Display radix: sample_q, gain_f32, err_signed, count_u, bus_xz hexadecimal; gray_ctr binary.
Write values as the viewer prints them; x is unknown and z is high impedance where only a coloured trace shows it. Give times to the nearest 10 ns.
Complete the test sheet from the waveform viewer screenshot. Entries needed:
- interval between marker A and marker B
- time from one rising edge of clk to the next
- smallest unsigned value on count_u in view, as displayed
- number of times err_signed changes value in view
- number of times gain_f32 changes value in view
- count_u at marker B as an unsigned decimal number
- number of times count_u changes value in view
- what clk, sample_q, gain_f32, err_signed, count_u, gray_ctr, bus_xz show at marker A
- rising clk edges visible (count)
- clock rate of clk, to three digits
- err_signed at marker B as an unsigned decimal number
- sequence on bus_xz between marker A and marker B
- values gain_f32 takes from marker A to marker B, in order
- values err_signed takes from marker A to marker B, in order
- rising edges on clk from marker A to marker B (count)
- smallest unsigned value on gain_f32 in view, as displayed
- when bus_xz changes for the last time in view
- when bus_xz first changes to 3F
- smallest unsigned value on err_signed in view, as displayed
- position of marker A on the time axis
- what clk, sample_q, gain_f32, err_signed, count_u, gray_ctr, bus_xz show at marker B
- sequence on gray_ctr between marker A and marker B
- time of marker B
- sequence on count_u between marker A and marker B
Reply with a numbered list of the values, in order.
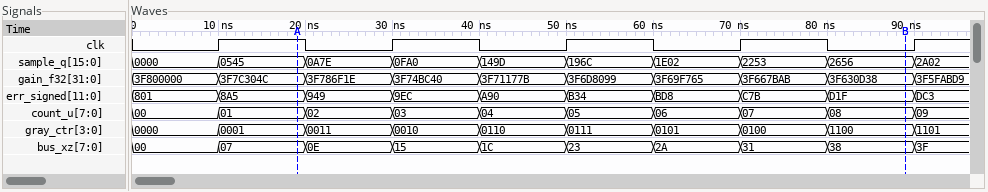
1. 70 ns
2. 20 ns
3. 00
4. 9
5. 9
6. 8
7. 9
8. clk=1, sample_q=0545, gain_f32=3F7C304C, err_signed=8A5, count_u=01, gray_ctr=0001, bus_xz=07
9. 5
10. 50.0 MHz
11. 3359
12. 07, 0E, 15, 1C, 23, 2A, 31, 38
13. 3F7C304C, 3F786F1E, 3F74BC40, 3F71177B, 3F6D8099, 3F69F765, 3F667BAB, 3F630D38
14. 8A5, 949, 9EC, A90, B34, BD8, C7B, D1F
15. 3
16. 3F5FABD9
17. 90 ns
18. 90 ns
19. 801
20. 20 ns
21. clk=0, sample_q=2656, gain_f32=3F630D38, err_signed=D1F, count_u=08, gray_ctr=1100, bus_xz=38
22. 0001, 0011, 0010, 0110, 0111, 0101, 0100, 1100
23. 90 ns
24. 01, 02, 03, 04, 05, 06, 07, 08
